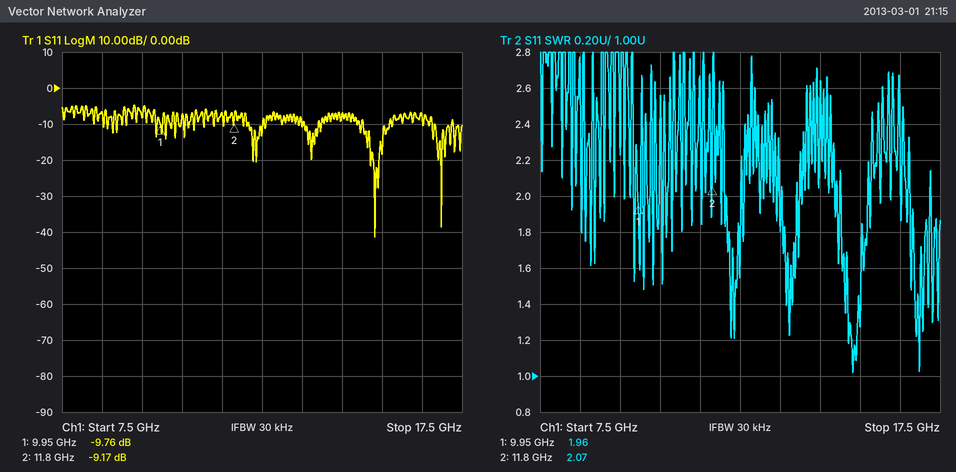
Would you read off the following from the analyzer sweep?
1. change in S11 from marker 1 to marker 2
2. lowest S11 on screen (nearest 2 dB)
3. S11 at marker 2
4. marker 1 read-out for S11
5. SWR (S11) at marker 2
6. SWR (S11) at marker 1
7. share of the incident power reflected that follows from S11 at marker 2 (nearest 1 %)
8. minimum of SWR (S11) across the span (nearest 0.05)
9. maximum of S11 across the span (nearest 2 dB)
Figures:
0.59 dB
-42 dB
-9.17 dB
-9.76 dB
2.07
1.96
12 %
1.00
-4 dB
